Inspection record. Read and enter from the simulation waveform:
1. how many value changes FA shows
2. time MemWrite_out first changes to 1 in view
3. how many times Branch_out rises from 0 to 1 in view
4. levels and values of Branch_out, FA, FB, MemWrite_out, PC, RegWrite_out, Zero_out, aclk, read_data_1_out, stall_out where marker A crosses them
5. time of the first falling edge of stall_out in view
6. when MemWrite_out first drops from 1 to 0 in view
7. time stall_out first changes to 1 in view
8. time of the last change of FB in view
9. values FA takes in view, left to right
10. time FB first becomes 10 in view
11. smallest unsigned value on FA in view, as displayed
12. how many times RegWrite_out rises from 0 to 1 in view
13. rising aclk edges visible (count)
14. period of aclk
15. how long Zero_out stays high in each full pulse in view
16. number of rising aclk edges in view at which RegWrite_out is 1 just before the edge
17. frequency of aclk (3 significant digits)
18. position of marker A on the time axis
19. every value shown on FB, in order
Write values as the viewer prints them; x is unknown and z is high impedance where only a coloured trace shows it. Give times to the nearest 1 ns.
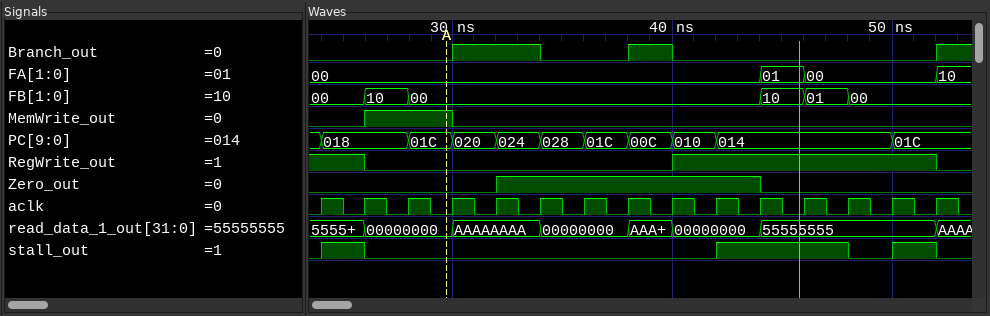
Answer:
3
26 ns
3
Branch_out=0, FA=00, FB=00, MemWrite_out=1, PC=01C, RegWrite_out=0, Zero_out=0, aclk=0, read_data_1_out=00000000, stall_out=0
26 ns
30 ns
24 ns
48 ns
00, 01, 00, 10
26 ns
00
1
15
2 ns
12 ns
8
500 MHz
30 ns
00, 10, 00, 10, 01, 00
